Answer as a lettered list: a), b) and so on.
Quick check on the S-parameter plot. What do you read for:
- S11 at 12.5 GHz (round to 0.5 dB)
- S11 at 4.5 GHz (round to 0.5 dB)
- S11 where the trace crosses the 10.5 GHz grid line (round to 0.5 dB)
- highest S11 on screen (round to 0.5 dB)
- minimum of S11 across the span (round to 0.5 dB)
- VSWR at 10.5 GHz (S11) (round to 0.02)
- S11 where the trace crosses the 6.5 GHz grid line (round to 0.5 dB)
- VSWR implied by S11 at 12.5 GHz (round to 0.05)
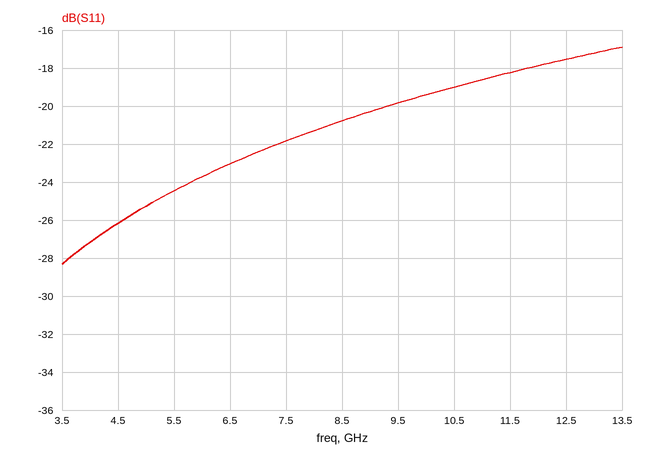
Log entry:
a) -17.5 dB
b) -26.0 dB
c) -19.0 dB
d) -17.0 dB
e) -28.5 dB
f) 1.26
g) -23.0 dB
h) 1.30
